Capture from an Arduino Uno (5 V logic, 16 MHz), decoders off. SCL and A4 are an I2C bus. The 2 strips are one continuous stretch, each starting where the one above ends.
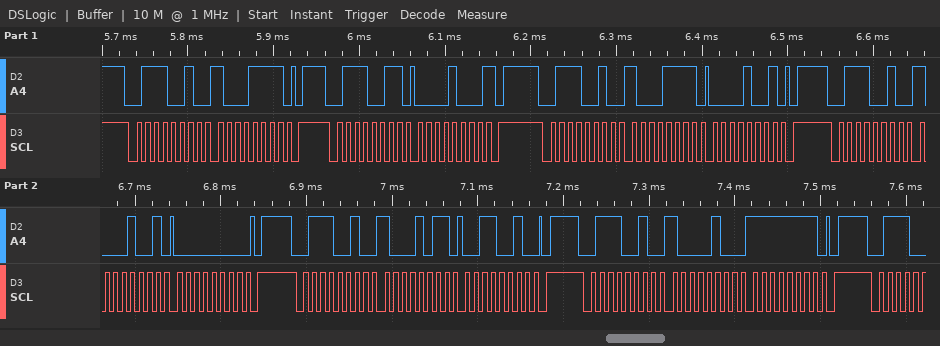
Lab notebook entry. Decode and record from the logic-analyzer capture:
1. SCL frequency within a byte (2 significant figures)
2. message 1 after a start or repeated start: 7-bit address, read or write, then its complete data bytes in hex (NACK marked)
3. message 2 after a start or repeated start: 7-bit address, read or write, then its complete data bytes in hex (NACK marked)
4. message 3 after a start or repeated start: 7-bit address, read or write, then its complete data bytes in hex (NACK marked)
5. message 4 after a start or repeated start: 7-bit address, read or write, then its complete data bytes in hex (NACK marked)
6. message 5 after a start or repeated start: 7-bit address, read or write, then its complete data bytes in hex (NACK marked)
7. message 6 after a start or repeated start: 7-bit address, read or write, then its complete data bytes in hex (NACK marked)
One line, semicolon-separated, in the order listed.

100 kHz; 0x39 write: 8F; 0x39 read: 08 NACK; 0x39 write: 8F 09; 0x39 write: 89 00; 0x39 write: 8B 32; 0x39 write: 84 FF
